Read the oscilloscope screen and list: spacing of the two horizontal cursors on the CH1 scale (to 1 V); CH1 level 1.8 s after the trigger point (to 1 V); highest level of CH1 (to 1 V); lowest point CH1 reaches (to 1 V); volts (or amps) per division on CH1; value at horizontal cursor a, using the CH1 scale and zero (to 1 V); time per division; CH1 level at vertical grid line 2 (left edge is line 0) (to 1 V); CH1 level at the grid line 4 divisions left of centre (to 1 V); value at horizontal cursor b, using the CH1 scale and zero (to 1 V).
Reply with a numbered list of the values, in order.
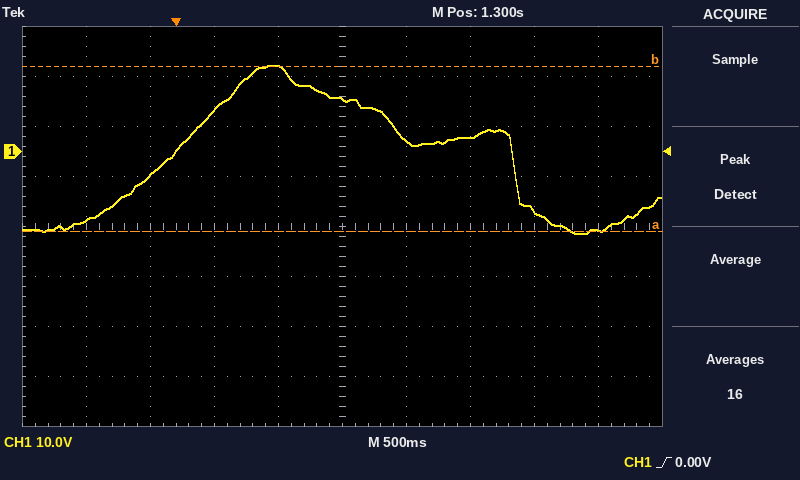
1. 33 V
2. 2 V
3. 17 V
4. -16 V
5. 10 V
6. -16 V
7. 500 ms
8. -5 V
9. -14 V
10. 17 V
